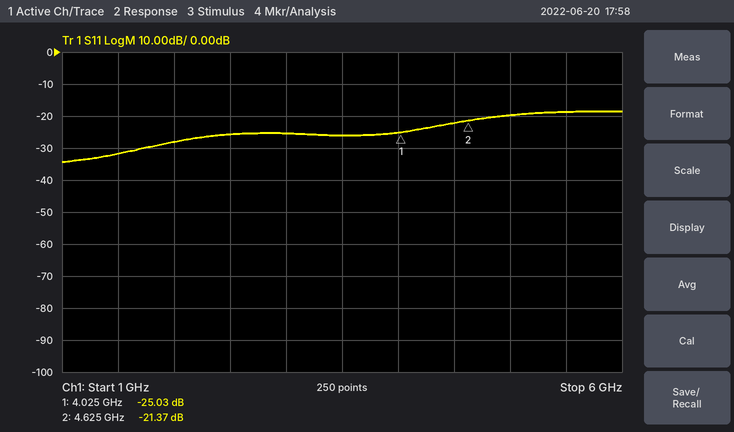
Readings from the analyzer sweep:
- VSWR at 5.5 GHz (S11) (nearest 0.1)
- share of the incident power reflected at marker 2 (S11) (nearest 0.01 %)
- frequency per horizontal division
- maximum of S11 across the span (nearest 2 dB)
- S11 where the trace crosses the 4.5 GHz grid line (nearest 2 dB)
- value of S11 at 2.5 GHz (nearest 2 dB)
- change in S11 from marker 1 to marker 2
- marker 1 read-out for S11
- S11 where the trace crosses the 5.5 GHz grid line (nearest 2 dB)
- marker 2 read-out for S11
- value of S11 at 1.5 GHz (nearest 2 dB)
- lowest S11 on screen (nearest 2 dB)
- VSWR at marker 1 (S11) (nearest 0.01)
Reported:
1.3
0.73 %
500 MHz
-18 dB
-22 dB
-26 dB
3.66 dB
-25.03 dB
-18 dB
-21.37 dB
-32 dB
-34 dB
1.12
